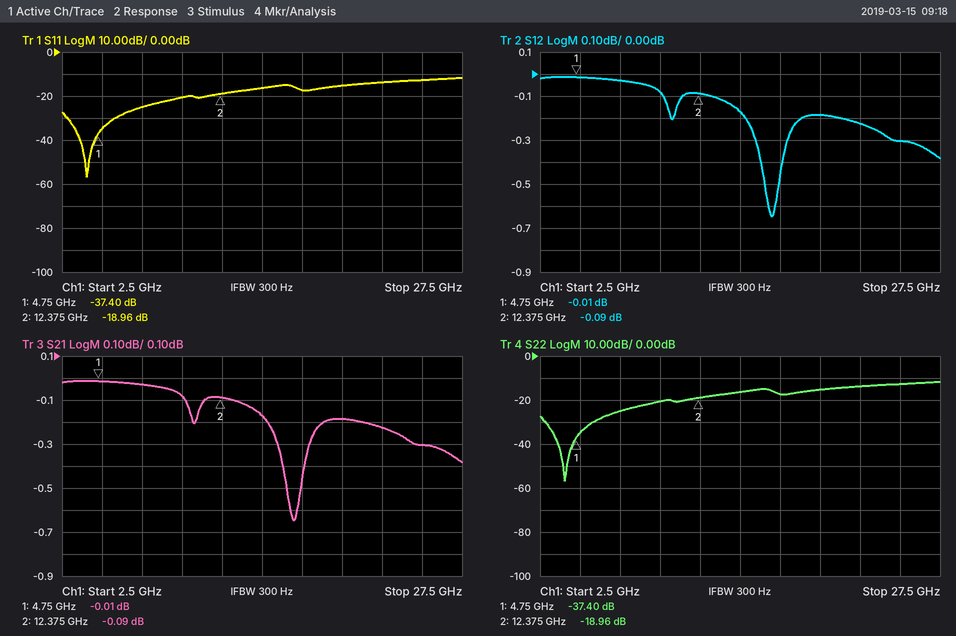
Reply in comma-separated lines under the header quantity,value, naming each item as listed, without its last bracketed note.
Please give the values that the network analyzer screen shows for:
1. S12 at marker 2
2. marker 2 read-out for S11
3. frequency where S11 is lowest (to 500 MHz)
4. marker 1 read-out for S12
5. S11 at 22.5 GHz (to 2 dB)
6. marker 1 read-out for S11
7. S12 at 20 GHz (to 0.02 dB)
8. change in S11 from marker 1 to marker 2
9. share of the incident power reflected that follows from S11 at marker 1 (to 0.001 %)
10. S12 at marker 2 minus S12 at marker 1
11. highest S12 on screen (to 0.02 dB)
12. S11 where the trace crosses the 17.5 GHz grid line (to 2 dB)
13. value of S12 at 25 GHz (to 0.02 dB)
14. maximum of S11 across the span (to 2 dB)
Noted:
quantity,value
S12 at marker 2,-0.09 dB
marker 2 read-out for S11,-18.96 dB
frequency where S11 is lowest,4.0 GHz
marker 1 read-out for S12,-0.01 dB
S11 at 22.5 GHz,-14 dB
marker 1 read-out for S11,-37.40 dB
S12 at 20 GHz,-0.18 dB
change in S11 from marker 1 to marker 2,18.44 dB
share of the incident power reflected that follows from S11 at marker 1,0.018 %
S12 at marker 2 minus S12 at marker 1,-0.08 dB
highest S12 on screen,-0.02 dB
S11 where the trace crosses the 17.5 GHz grid line,-18 dB
value of S12 at 25 GHz,-0.30 dB
maximum of S11 across the span,-12 dB
